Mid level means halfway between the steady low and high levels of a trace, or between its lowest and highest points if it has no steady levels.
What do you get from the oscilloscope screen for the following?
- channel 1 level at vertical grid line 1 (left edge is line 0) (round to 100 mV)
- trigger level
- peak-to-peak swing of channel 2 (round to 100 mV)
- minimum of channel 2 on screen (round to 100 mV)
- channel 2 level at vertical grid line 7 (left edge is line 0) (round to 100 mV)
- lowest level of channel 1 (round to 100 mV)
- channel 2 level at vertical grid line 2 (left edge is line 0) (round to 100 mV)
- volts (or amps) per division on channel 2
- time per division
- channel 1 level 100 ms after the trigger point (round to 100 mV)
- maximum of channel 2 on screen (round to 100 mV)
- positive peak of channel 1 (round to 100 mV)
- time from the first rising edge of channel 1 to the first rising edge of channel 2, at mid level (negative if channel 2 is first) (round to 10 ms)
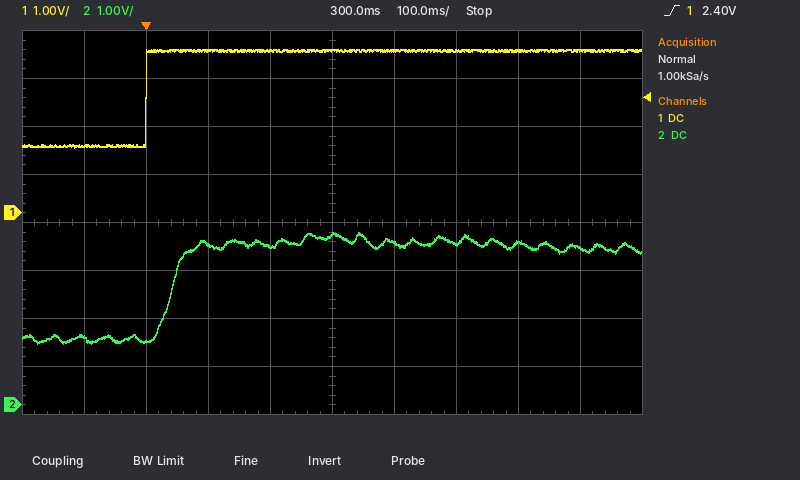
1.4 V
2.40 V
2.3 V
1.3 V
3.4 V
1.4 V
1.3 V
1 V
100 ms
3.4 V
3.6 V
3.4 V
+40 ms
